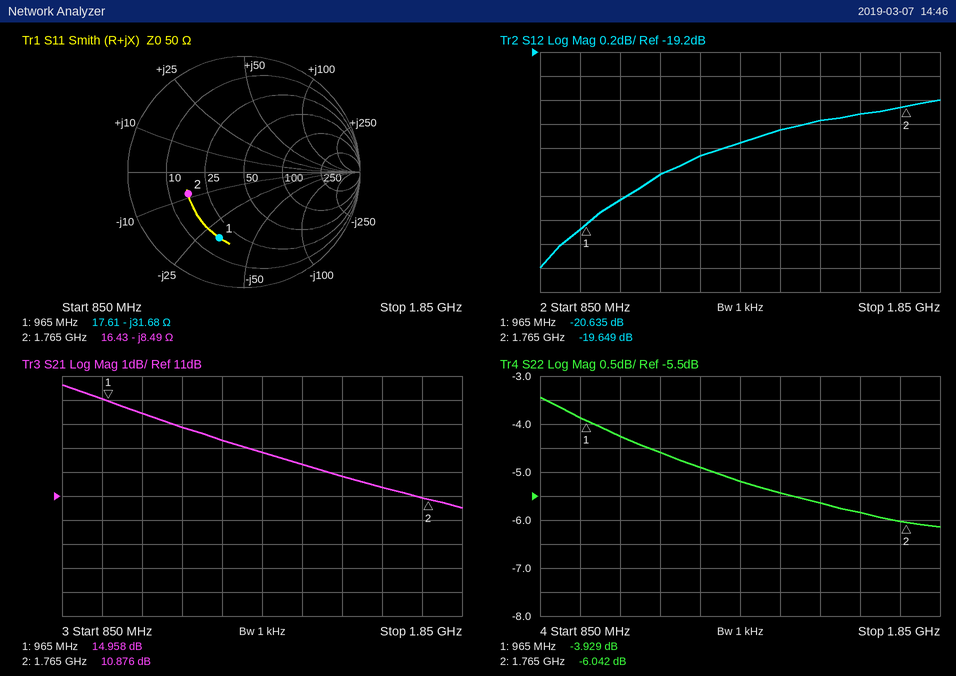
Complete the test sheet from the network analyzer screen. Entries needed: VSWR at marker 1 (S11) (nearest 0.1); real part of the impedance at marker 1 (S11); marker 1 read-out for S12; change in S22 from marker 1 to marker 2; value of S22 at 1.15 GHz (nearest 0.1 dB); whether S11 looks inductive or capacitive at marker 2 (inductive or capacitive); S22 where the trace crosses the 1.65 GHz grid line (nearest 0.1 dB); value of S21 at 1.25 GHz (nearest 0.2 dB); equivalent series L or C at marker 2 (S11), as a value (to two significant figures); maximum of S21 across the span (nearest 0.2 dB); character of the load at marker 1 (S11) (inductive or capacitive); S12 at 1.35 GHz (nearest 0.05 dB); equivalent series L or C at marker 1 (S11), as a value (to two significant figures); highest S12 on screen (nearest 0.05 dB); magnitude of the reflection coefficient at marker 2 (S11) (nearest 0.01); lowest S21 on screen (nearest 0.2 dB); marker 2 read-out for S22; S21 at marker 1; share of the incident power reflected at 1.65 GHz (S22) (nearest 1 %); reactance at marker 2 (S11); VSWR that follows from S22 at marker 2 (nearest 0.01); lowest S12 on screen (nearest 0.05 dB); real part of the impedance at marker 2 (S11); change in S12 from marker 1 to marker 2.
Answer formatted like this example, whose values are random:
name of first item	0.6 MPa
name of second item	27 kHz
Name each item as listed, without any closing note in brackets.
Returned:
VSWR at marker 1 (S11)	4.1
real part of the impedance at marker 1	17.61 Ω
marker 1 read-out for S12	-20.635 dB
change in S22 from marker 1 to marker 2	-2.113 dB
value of S22 at 1.15 GHz	-4.6 dB
whether S11 looks inductive or capacitive at marker 2	capacitive
S22 where the trace crosses the 1.65 GHz grid line	-5.8 dB
value of S21 at 1.25 GHz	13.4 dB
equivalent series L or C at marker 2 (S11), as a value	11 pF
maximum of S21 across the span	15.6 dB
character of the load at marker 1 (S11)	capacitive
S12 at 1.35 GHz	-19.95 dB
equivalent series L or C at marker 1 (S11), as a value	5.2 pF
highest S12 on screen	-19.60 dB
magnitude of the reflection coefficient at marker 2 (S11)	0.52
lowest S21 on screen	10.6 dB
marker 2 read-out for S22	-6.042 dB
S21 at marker 1	14.958 dB
share of the incident power reflected at 1.65 GHz (S22)	26 %
reactance at marker 2	-8.49 Ω
VSWR that follows from S22 at marker 2	2.99
lowest S12 on screen	-21.00 dB
real part of the impedance at marker 2	16.43 Ω
change in S12 from marker 1 to marker 2	0.986 dB
